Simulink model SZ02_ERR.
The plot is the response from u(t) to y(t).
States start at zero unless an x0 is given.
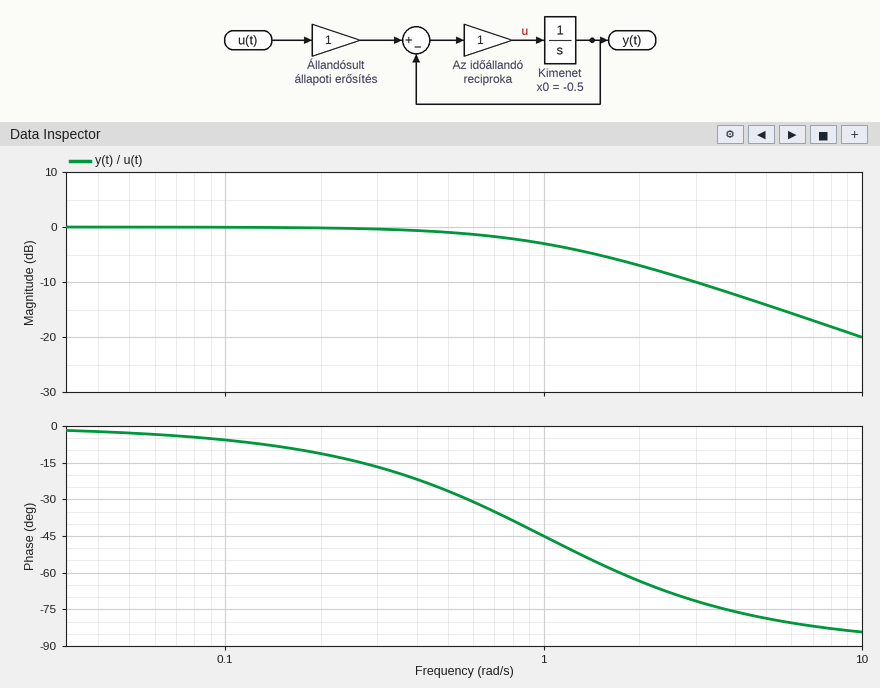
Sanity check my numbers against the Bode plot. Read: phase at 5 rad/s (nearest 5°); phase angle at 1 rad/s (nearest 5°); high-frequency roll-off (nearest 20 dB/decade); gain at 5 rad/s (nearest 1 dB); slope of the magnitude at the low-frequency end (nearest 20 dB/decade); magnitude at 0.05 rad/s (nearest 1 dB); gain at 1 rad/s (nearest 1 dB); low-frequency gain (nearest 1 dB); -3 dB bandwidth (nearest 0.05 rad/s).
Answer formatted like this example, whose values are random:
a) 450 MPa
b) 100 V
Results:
a) -80°
b) -45°
c) -20 dB/decade
d) -14 dB
e) 0 dB/decade
f) 0 dB
g) -3 dB
h) 0 dB
i) 1.00 rad/s
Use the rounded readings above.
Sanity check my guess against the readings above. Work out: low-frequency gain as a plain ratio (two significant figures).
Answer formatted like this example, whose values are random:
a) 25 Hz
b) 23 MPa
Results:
a) 1.0
